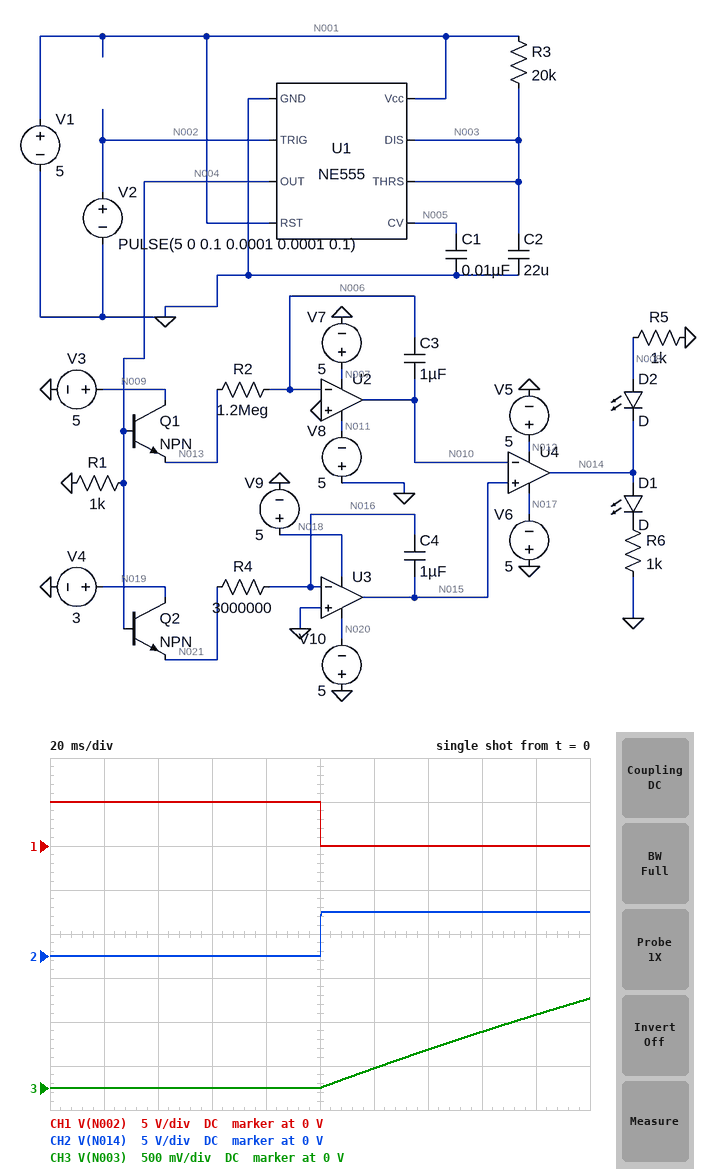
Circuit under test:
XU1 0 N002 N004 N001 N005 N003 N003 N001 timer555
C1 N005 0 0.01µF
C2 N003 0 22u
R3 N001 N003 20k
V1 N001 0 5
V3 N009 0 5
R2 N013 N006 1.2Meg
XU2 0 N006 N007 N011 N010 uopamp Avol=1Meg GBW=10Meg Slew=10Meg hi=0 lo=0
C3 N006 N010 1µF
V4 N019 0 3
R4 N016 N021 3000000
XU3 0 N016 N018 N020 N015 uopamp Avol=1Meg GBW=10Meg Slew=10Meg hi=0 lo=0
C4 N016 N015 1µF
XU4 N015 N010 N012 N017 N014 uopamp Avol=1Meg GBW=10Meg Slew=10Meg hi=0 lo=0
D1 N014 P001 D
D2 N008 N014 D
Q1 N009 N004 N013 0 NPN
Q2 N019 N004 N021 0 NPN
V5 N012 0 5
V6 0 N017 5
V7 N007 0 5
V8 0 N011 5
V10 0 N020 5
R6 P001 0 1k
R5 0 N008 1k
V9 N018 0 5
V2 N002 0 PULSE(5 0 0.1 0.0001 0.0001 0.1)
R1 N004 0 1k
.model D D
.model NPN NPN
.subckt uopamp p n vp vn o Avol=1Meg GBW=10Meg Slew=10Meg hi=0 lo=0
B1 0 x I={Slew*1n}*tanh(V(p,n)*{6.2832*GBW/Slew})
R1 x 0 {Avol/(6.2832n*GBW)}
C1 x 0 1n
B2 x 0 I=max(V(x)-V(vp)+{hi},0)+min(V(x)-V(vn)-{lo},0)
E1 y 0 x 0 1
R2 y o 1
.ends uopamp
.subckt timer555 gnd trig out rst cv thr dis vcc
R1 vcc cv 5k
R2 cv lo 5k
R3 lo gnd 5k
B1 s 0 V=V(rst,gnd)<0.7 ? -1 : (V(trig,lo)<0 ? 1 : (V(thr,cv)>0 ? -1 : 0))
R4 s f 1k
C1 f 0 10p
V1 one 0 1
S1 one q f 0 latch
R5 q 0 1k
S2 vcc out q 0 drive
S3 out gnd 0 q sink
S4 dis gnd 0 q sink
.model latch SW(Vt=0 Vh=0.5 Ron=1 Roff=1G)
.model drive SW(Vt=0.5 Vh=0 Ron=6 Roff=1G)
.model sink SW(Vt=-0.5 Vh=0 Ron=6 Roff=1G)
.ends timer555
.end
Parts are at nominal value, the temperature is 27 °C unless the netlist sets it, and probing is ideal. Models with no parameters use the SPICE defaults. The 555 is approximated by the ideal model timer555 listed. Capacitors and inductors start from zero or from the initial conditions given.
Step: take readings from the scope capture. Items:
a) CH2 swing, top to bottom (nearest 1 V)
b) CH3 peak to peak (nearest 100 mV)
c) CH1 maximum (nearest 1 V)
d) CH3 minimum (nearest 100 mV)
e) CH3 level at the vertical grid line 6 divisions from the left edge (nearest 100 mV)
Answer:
5 V
1.0 V
5 V
0 V
200 mV
